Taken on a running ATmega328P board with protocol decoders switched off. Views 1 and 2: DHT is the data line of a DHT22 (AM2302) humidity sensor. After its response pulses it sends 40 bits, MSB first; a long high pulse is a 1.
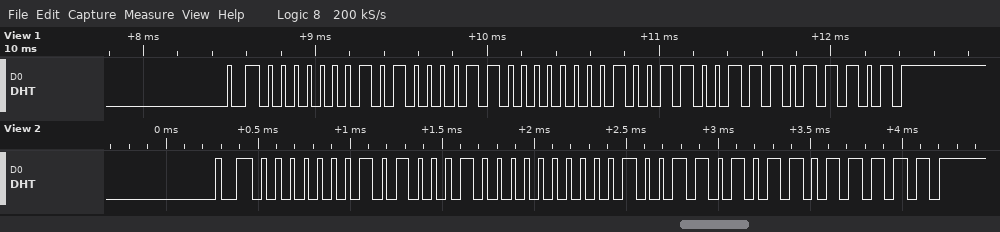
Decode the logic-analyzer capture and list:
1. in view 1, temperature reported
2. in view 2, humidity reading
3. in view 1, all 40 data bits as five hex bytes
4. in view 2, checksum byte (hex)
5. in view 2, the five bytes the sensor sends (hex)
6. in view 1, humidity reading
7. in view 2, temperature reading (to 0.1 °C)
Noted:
15.3 °C
32.4 %
01 43 00 99 DD
0xDF
01 44 00 9A DF
32.3 %
15.4 °C
